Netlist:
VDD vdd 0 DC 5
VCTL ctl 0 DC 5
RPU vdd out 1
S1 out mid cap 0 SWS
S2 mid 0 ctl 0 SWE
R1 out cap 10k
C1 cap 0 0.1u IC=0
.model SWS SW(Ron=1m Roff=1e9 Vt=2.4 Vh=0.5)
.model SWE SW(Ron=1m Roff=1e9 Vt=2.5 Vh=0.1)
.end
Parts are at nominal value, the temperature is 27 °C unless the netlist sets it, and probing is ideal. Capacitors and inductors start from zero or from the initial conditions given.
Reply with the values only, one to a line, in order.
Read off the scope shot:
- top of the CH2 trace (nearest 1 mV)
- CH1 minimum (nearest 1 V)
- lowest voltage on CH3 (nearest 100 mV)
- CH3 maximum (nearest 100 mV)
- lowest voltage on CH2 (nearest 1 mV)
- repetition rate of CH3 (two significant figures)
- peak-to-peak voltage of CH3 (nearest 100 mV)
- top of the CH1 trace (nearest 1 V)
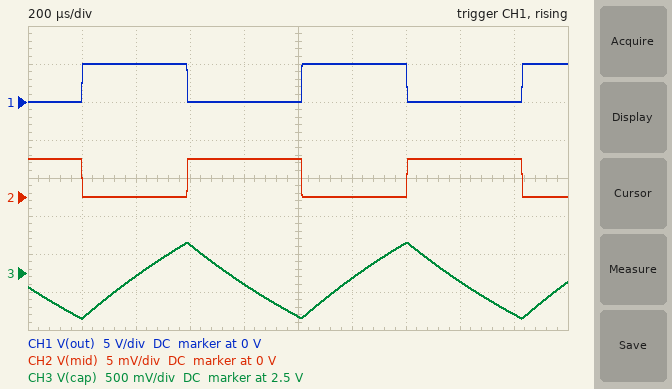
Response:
5 mV
0 V
1.9 V
2.9 V
0 V
1.2 kHz
1.0 V
5 V
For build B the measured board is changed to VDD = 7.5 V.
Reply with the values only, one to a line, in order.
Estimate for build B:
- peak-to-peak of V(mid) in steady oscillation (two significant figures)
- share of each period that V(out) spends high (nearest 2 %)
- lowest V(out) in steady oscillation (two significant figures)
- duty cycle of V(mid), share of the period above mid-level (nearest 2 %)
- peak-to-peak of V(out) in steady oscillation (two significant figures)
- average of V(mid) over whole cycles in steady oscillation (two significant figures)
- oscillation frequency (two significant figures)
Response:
7.5 mV
32 %
15 mV
68 %
7.5 V
5.1 mV
1.6 kHz
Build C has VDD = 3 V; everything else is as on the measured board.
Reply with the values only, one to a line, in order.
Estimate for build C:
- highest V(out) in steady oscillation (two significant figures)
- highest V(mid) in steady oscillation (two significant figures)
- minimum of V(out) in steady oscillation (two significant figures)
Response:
3.0 V
3.0 mV
6.0 mV
